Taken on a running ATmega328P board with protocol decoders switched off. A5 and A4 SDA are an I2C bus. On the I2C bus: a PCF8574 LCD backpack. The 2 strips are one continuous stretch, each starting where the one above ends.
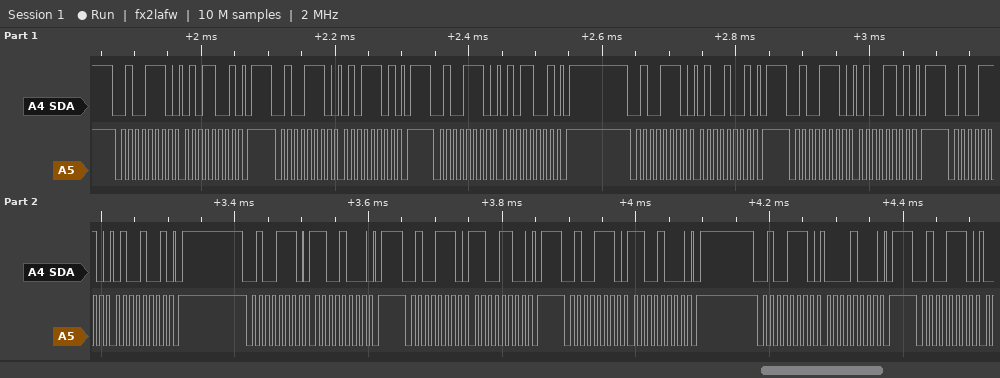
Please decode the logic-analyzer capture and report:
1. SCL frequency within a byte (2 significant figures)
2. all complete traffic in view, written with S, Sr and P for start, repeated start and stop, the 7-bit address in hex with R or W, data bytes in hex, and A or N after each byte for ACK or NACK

100 kHz
S 27W A 59 A P S 27W A 5D A P S 27W A 59 A P S 27W A 49 A P S 27W A 4D A P S 27W A 49 A P S 27W A C8 A P S 27W A CC A P S 27W A C8 A P S 27W A 08 A P S 27W A
